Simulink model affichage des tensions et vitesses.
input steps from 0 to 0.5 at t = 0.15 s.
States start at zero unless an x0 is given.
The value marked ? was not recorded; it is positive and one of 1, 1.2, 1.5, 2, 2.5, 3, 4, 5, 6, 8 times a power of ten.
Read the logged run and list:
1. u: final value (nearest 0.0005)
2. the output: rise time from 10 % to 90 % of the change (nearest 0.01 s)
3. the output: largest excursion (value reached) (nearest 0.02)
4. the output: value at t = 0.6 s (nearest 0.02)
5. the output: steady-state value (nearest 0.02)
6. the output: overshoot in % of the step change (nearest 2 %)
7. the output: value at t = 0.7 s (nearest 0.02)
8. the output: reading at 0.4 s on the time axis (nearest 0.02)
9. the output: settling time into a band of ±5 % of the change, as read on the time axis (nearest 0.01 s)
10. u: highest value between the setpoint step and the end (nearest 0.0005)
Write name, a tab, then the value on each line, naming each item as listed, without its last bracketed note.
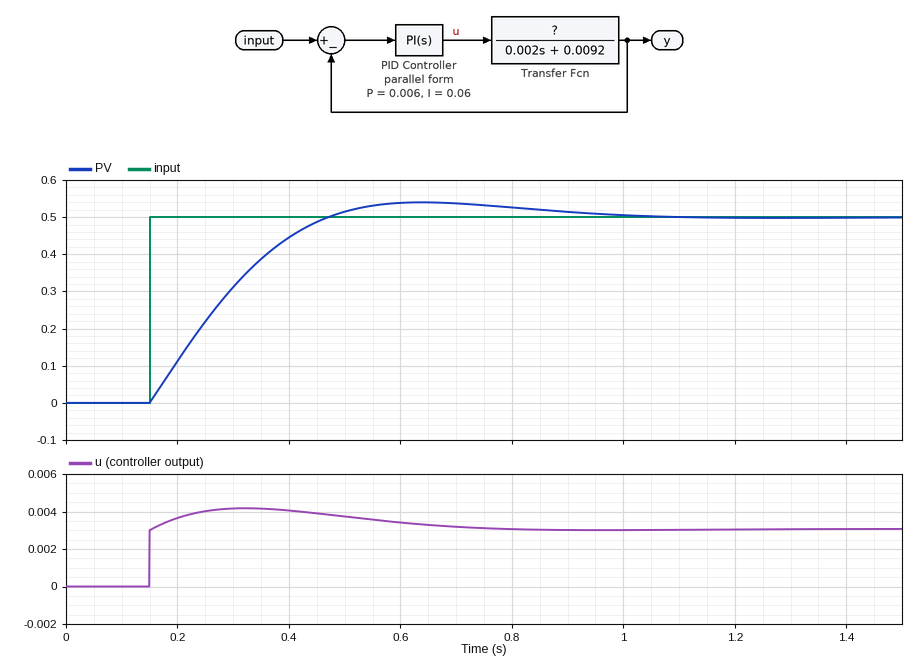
u: final value	0.0030
the output: rise time from 10 % to 90 % of the change	0.23 s
the output: largest excursion (value reached)	0.54
the output: value at t = 0.6 s	0.54
the output: steady-state value	0.50
the output: overshoot in % of the step change	8 %
the output: value at t = 0.7 s	0.54
the output: reading at 0.4 s on the time axis	0.44
the output: settling time into a band of ±5 % of the change, as read on the time axis	0.81 s
u: highest value between the setpoint step and the end	0.0040
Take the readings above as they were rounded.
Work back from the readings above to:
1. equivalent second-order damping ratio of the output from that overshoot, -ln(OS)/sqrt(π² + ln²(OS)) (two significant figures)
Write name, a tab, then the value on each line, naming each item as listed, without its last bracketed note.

equivalent second-order damping ratio of the output from that overshoot, -ln(OS)/sqrt(π² + ln²(OS))	0.63
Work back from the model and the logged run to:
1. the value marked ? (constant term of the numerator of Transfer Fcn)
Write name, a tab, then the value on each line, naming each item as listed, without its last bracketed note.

the value marked ?	1.5
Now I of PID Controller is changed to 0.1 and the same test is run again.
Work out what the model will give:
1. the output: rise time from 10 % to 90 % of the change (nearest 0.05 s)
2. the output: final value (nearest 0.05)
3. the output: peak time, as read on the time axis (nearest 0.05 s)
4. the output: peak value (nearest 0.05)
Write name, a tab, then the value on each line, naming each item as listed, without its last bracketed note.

the output: rise time from 10 % to 90 % of the change	0.15 s
the output: final value	0.50
the output: peak time, as read on the time axis	0.50 s
the output: peak value	0.60
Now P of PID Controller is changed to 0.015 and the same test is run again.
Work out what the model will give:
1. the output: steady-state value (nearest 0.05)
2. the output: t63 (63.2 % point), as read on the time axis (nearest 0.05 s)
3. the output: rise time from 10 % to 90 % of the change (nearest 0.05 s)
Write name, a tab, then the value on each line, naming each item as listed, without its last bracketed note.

the output: steady-state value	0.50
the output: t63 (63.2 % point), as read on the time axis	0.25 s
the output: rise time from 10 % to 90 % of the change	0.20 s
